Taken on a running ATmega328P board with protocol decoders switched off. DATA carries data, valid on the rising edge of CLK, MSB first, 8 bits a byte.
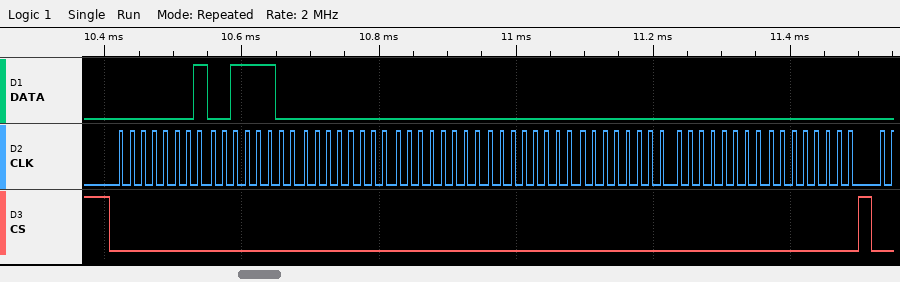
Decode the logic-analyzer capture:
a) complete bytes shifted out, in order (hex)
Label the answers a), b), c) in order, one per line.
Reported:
a) 01 3C 00 00 00 00 00 00
